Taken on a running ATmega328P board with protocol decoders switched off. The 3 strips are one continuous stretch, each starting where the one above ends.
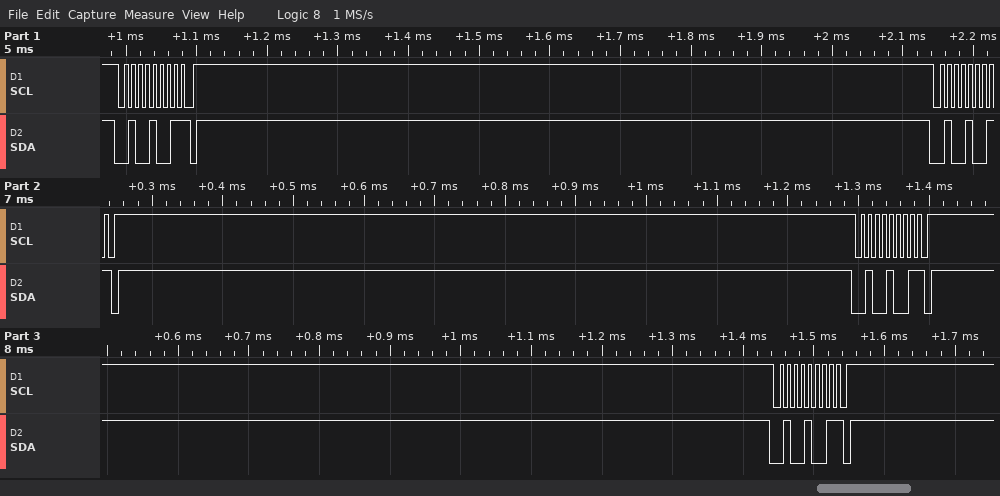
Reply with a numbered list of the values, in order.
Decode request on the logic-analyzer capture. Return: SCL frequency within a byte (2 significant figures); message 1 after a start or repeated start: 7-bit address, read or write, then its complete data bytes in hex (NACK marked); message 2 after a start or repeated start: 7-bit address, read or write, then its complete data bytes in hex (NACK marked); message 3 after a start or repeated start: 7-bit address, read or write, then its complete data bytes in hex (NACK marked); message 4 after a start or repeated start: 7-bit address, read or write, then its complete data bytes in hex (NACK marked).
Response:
1. 100 kHz
2. 0x24 read NACK
3. 0x24 read NACK
4. 0x24 read NACK
5. 0x24 read NACK
